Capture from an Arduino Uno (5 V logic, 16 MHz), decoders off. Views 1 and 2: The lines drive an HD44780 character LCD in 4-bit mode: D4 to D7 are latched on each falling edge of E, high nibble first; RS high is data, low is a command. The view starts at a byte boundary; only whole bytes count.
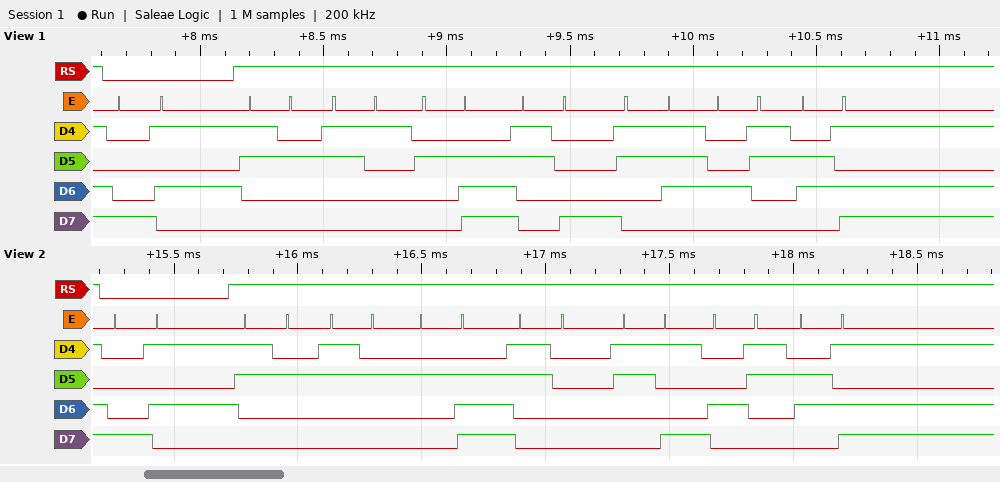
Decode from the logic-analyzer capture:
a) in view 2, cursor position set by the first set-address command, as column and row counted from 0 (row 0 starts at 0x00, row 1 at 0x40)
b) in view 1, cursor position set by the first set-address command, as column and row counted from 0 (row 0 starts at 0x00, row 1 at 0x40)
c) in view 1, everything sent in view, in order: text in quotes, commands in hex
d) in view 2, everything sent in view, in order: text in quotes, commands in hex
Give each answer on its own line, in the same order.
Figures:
column 5, row 0
column 5, row 0
0x85 "21.87Cm"
0x85 "22.09Cm"
